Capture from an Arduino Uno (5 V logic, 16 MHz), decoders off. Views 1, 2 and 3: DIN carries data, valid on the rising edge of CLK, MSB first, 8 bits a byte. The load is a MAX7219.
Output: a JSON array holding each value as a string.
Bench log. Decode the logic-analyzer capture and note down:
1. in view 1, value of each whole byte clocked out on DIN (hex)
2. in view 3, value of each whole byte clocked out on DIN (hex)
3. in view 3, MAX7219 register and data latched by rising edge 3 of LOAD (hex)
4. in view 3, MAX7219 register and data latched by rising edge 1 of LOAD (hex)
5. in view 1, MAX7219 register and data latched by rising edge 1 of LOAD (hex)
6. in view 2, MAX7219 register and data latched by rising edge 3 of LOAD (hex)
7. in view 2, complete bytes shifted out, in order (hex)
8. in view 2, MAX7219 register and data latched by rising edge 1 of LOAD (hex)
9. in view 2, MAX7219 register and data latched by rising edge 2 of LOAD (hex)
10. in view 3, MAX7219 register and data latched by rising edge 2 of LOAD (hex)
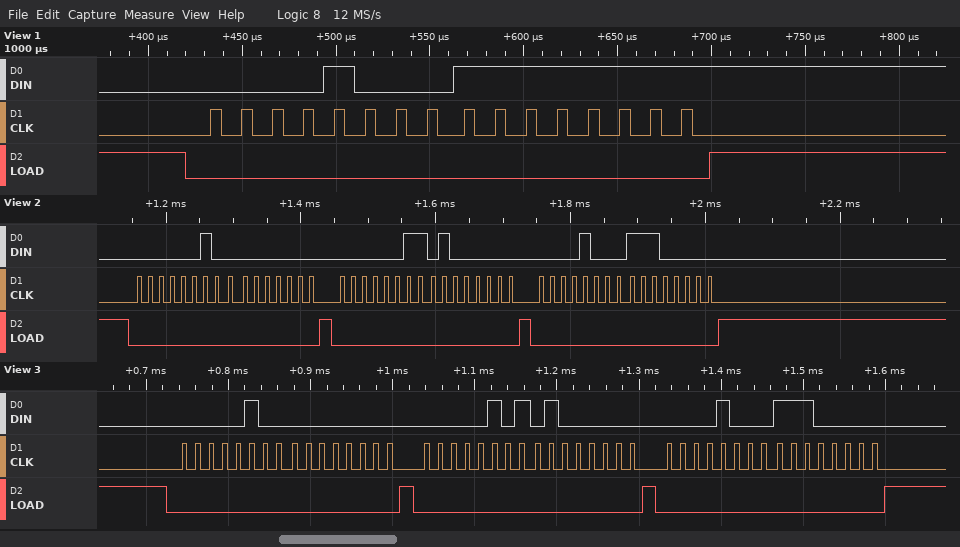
["0x08 0xFF", "04 00 05 40 08 E0", "register 0x8, data 0xE0", "register 0x4, data 0x00", "register 0x8, data 0xFF", "register 0x8, data 0xE0", "02 00 03 40 08 E0", "register 0x2, data 0x00", "register 0x3, data 0x40", "register 0x5, data 0x40"]
